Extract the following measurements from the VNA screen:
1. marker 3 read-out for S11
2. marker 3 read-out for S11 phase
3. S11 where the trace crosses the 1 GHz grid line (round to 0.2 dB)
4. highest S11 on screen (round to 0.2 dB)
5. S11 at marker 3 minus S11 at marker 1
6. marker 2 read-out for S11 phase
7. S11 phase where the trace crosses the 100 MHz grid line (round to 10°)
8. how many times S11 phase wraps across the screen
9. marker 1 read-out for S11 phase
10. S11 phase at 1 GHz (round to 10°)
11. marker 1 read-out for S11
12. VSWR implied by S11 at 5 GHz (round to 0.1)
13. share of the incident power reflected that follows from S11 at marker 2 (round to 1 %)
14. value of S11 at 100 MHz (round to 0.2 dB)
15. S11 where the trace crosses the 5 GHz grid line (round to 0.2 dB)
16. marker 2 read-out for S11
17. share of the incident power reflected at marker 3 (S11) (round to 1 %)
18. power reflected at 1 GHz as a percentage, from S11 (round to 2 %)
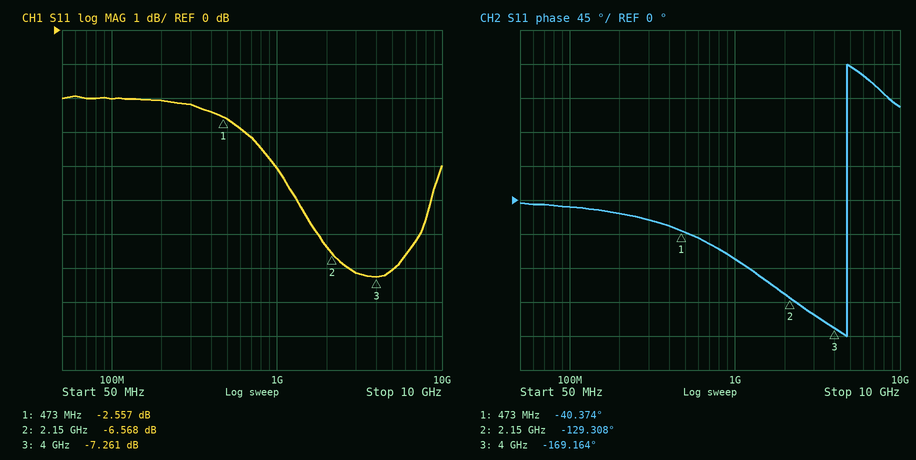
-7.261 dB
-169.164°
-4.0 dB
-2.0 dB
-4.704 dB
-129.308°
-10°
1
-40.374°
-80°
-2.557 dB
2.6
22 %
-2.0 dB
-7.0 dB
-6.568 dB
19 %
40 %
